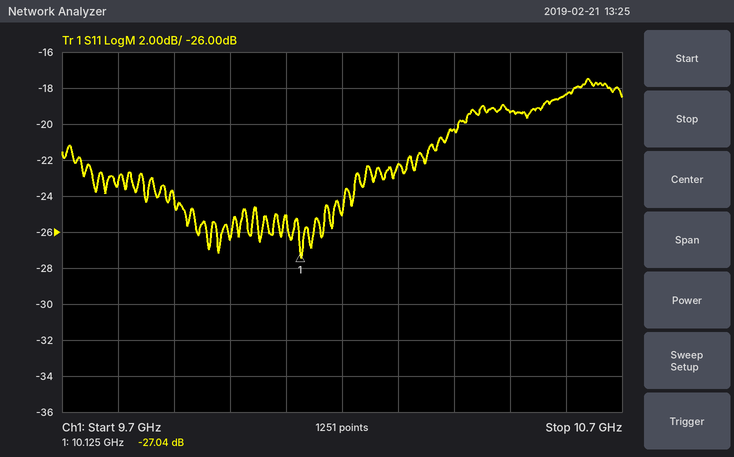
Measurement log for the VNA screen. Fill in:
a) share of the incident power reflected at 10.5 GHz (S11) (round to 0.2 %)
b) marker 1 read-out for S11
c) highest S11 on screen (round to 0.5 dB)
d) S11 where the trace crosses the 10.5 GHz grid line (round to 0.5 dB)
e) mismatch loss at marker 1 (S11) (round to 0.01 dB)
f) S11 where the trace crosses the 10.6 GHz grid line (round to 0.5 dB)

1.2 %
-27.04 dB
-17.5 dB
-19.5 dB
0.01 dB
-18.5 dB
